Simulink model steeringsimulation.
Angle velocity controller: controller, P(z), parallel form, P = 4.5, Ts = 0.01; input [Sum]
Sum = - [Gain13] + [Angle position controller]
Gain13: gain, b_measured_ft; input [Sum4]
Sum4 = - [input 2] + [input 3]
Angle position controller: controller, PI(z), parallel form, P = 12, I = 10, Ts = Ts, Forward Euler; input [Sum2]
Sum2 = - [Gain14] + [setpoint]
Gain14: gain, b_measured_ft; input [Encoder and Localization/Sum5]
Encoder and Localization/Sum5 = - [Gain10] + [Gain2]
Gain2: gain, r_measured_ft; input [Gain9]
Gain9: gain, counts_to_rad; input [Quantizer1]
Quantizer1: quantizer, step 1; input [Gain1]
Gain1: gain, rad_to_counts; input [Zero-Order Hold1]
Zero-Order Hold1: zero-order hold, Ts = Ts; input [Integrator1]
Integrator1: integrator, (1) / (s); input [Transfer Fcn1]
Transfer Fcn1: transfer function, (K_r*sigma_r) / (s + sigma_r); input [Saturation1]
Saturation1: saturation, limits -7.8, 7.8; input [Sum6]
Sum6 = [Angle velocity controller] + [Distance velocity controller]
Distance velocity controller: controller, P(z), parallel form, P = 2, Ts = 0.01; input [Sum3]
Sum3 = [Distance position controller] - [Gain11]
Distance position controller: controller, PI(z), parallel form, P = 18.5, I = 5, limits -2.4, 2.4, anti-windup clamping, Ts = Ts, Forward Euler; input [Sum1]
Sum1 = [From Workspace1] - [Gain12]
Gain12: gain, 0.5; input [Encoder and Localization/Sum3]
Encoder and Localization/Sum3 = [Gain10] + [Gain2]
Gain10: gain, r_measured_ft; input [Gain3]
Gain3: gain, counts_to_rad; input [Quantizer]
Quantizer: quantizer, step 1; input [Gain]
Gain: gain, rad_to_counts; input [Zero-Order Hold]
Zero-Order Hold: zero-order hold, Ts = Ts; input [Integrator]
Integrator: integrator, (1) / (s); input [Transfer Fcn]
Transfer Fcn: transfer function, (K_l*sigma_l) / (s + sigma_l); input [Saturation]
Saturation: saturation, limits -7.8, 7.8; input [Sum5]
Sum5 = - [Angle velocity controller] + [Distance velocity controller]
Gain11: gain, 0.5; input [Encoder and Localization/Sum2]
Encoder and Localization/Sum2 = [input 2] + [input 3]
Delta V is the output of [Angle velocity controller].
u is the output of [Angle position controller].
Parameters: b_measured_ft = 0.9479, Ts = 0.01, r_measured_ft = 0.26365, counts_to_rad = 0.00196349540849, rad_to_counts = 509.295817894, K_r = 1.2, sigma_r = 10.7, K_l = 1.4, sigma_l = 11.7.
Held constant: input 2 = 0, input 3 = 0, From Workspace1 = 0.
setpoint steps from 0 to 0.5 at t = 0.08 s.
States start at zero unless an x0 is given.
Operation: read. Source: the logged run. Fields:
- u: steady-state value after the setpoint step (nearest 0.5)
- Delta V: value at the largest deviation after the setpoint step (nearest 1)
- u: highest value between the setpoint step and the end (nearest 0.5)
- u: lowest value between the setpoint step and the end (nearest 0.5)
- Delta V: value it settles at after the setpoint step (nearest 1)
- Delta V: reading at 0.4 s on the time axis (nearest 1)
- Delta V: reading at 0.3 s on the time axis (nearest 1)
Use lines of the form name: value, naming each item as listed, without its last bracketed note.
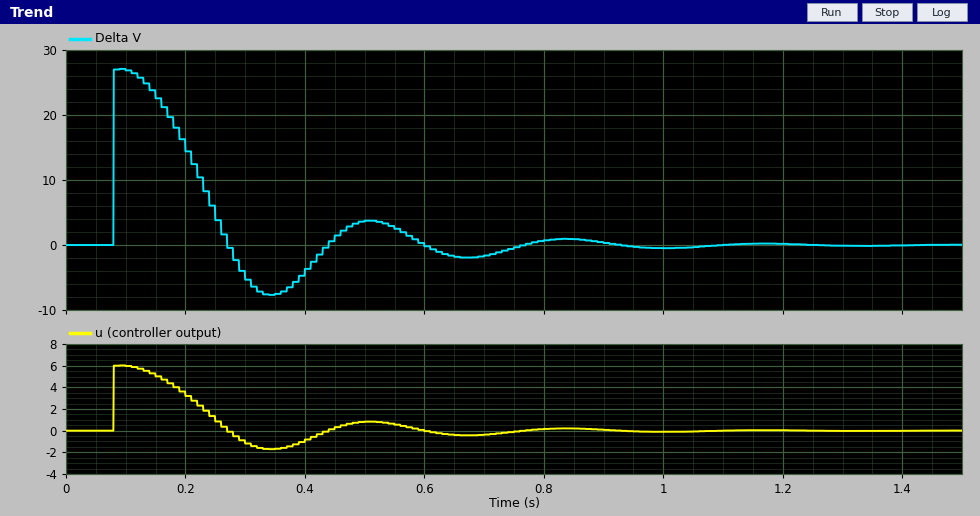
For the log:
u: steady-state value after the setpoint step: 0.0
Delta V: value at the largest deviation after the setpoint step: 27
u: highest value between the setpoint step and the end: 6.0
u: lowest value between the setpoint step and the end: -1.5
Delta V: value it settles at after the setpoint step: 0
Delta V: reading at 0.4 s on the time axis: -4
Delta V: reading at 0.3 s on the time axis: -5
